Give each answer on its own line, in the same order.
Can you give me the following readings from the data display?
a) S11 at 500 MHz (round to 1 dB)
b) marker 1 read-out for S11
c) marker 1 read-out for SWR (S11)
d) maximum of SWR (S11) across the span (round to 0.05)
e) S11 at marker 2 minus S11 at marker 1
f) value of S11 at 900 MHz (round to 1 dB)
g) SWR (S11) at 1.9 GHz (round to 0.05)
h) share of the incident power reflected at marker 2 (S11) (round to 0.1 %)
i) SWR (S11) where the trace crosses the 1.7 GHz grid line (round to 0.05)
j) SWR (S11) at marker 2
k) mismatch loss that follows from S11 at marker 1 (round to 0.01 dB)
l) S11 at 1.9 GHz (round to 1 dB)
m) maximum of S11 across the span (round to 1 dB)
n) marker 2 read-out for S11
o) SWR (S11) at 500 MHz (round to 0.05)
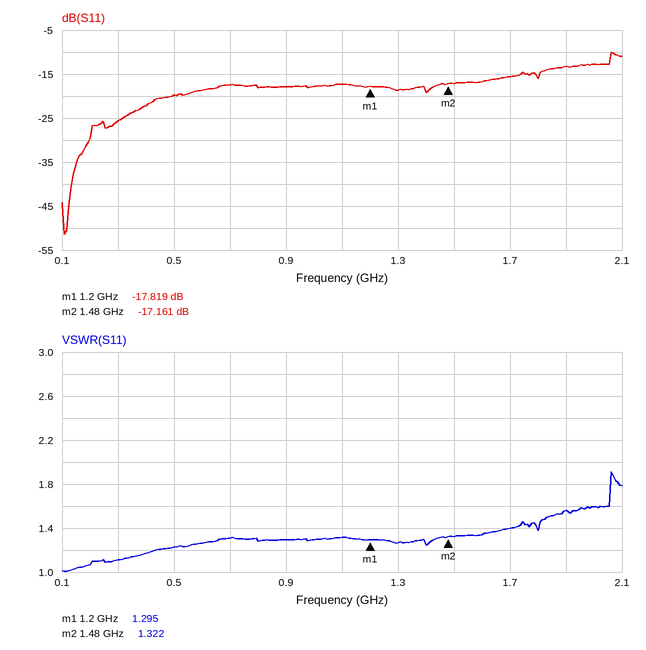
-20 dB
-17.819 dB
1.295
1.90
0.658 dB
-18 dB
1.55
1.9 %
1.40
1.322
0.07 dB
-13 dB
-10 dB
-17.161 dB
1.25
